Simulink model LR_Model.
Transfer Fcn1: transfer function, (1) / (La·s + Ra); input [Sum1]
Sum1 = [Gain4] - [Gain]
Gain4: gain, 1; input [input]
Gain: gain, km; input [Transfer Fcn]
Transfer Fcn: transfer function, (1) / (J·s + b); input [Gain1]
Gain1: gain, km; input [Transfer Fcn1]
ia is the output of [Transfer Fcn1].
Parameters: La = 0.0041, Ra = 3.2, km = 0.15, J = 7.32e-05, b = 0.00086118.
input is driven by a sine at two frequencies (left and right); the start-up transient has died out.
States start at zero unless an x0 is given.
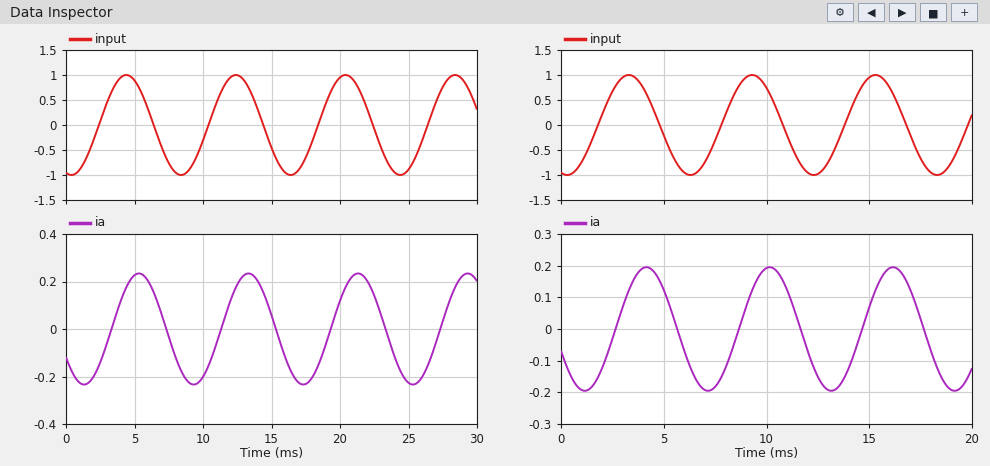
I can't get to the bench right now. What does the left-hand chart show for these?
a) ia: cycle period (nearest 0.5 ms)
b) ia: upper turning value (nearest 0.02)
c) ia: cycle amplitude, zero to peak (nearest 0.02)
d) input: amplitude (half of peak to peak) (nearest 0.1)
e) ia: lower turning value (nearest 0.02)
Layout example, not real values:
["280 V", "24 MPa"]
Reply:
["8.0 ms", "0.24", "0.24", "1.0", "-0.24"]
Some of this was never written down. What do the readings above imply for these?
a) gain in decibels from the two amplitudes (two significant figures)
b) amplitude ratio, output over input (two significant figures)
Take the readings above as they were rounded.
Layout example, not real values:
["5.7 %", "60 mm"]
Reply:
["-12 dB", "0.24"]
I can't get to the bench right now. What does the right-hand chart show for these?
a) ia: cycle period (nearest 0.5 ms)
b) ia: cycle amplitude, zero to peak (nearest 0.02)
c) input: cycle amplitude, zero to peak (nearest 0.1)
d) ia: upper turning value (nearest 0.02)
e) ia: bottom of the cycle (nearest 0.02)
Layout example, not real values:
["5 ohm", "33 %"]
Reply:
["6.0 ms", "0.20", "1.0", "0.20", "-0.20"]
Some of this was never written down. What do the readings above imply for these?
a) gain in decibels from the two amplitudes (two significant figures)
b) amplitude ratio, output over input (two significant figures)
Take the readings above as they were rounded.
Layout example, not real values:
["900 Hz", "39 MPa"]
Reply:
["-14 dB", "0.20"]
